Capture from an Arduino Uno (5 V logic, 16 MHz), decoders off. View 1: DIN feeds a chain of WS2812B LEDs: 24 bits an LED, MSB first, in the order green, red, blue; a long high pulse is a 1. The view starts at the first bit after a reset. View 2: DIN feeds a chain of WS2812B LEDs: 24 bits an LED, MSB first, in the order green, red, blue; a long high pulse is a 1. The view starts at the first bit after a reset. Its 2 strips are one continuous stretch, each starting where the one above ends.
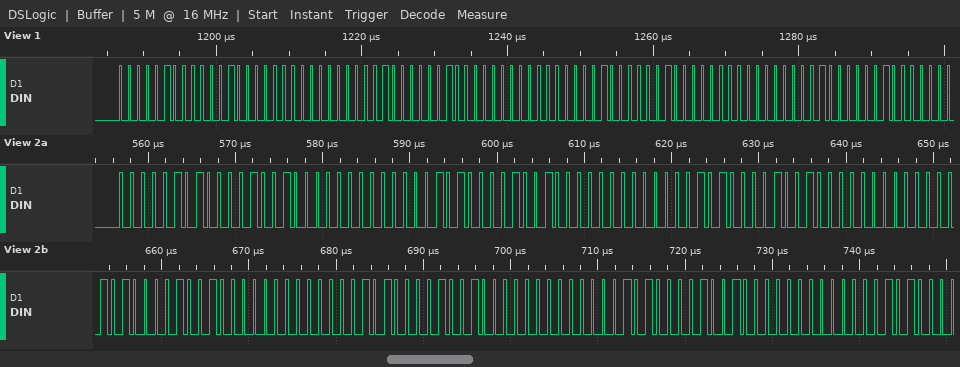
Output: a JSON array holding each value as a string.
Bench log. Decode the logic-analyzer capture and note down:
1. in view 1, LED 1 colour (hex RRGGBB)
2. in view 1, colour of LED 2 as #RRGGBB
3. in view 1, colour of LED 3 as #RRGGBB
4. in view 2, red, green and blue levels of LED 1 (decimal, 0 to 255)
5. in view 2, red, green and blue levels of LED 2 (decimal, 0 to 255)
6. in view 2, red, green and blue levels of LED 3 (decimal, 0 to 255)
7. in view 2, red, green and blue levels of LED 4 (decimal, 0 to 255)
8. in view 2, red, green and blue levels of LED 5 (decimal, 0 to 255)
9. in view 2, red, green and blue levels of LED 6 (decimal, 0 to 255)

["#080400", "#080400", "#080400", "9, 5, 0", "9, 5, 0", "9, 5, 0", "9, 5, 0", "9, 5, 0", "9, 5, 0"]
